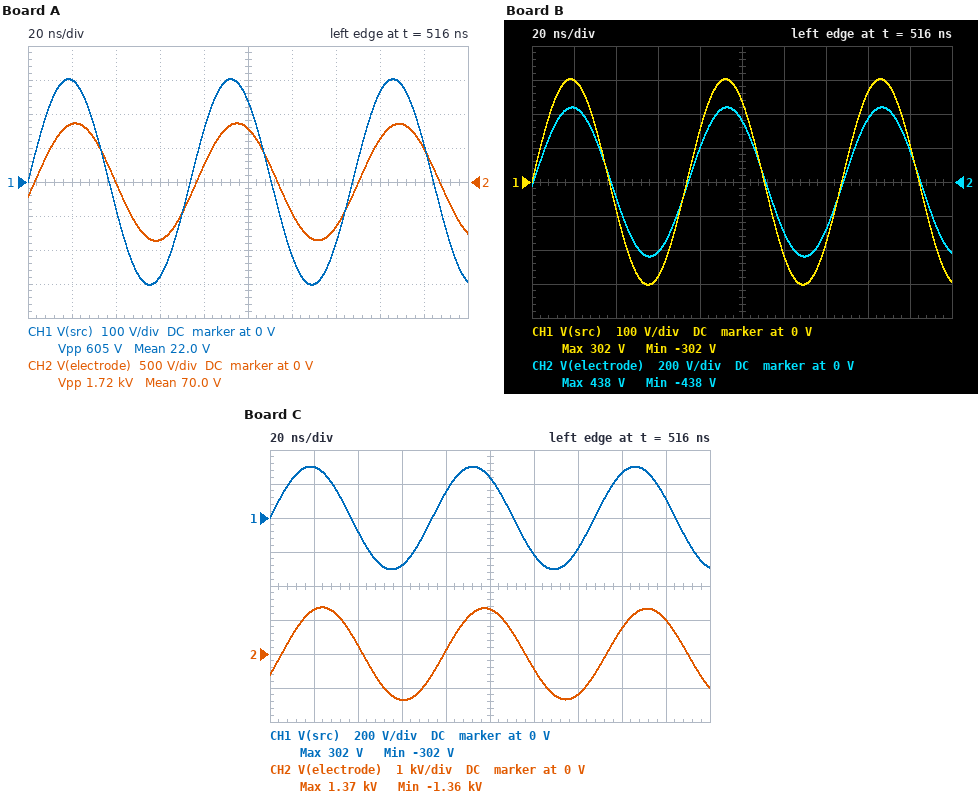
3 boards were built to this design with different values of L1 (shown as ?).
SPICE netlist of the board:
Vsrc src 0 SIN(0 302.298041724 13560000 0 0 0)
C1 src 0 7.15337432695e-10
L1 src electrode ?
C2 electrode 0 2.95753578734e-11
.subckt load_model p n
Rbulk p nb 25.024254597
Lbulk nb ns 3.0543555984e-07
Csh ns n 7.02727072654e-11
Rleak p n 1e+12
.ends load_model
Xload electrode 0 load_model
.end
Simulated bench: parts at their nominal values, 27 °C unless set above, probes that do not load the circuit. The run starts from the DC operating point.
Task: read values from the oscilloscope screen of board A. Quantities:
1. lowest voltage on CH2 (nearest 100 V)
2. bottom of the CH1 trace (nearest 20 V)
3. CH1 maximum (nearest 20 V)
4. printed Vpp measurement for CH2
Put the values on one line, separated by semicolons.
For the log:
-900 V; -300 V; 300 V; 1.72 kV
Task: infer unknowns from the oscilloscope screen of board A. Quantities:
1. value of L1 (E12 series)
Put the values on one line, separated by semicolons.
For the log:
820 nH
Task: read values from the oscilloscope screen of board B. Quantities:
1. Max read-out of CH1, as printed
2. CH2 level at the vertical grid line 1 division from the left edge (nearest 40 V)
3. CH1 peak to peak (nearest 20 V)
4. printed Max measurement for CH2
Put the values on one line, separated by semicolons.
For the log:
302 V; 440 V; 600 V; 438 V
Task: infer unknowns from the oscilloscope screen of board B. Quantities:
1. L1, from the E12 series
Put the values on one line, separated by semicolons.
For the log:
390 nH
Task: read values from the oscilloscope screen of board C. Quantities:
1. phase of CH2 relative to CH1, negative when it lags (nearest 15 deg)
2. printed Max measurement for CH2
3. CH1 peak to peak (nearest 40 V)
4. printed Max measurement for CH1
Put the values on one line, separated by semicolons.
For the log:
-30 deg; 1.37 kV; 600 V; 302 V
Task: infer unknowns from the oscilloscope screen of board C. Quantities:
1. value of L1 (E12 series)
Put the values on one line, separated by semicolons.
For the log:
1 µH
